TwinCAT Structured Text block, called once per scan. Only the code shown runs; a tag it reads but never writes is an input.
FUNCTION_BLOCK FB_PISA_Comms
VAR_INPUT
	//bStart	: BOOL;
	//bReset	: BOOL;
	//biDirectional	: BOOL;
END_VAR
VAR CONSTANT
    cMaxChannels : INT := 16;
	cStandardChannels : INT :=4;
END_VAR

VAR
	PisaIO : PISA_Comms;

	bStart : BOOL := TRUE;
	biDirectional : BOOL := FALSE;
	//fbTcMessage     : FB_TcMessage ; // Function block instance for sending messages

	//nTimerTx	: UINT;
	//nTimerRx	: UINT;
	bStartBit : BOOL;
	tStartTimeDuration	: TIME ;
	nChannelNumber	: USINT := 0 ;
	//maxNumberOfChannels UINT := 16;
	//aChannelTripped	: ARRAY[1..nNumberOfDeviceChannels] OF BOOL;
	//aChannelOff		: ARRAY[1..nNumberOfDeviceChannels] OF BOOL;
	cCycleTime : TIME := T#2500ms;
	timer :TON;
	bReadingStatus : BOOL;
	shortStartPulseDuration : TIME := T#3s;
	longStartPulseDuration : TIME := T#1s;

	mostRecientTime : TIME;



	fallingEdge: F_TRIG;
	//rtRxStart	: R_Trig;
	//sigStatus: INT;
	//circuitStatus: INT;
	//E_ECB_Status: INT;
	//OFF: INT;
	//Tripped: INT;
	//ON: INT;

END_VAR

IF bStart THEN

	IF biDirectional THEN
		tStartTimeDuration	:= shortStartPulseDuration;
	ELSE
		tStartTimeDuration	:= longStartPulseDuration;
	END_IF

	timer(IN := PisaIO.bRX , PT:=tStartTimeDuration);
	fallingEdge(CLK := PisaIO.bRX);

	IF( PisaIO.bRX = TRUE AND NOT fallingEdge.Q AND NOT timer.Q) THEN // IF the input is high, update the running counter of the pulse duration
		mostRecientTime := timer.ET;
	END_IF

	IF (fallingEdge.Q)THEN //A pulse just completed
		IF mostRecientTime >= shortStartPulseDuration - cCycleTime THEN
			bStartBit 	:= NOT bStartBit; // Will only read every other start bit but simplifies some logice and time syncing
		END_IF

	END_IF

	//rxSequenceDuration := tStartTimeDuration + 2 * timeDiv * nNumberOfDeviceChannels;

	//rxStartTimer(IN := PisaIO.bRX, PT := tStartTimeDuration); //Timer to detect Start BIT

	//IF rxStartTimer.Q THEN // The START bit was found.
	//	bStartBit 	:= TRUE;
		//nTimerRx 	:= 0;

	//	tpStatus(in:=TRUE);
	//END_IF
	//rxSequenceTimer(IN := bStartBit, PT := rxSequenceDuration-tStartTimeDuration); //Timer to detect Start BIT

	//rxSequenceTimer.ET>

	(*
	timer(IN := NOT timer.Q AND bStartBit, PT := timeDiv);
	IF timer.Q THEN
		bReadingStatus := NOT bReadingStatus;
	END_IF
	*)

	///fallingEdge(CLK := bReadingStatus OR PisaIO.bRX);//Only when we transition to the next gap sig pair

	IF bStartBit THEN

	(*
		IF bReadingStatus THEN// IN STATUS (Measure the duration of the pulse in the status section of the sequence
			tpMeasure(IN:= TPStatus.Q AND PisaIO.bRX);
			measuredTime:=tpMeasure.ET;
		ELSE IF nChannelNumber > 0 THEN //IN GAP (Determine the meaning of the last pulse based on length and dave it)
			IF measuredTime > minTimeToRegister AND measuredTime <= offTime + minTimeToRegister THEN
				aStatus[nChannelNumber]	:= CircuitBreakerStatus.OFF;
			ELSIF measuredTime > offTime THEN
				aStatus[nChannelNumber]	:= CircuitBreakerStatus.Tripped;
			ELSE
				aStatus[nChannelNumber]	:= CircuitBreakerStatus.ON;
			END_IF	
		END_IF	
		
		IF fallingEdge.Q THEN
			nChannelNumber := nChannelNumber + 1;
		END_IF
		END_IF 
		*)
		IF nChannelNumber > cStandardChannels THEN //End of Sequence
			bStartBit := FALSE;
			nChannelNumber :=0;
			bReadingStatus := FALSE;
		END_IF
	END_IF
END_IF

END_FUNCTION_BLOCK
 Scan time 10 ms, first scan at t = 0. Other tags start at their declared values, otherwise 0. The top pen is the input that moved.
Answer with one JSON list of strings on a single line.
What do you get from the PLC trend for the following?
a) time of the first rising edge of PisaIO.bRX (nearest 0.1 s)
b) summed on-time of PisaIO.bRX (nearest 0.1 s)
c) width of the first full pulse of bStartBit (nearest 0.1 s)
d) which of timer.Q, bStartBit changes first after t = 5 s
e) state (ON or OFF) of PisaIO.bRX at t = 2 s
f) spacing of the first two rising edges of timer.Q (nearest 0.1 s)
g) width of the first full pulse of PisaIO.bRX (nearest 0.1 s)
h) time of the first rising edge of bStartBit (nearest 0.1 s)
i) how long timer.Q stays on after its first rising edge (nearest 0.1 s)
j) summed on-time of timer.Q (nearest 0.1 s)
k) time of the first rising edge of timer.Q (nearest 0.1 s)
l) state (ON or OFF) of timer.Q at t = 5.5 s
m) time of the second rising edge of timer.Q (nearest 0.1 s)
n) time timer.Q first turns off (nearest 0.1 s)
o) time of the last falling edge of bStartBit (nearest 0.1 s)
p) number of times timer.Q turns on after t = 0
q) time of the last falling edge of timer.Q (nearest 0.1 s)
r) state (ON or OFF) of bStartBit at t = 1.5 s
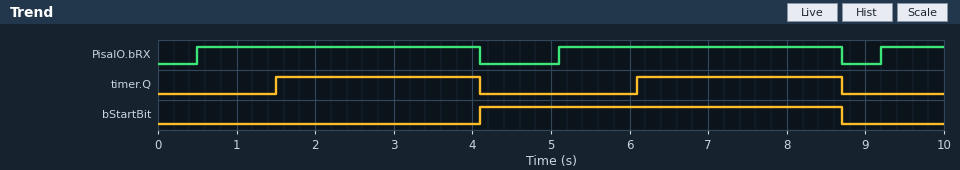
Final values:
["0.5 s", "8.0 s", "4.6 s", "timer.Q", "ON", "4.6 s", "3.6 s", "4.1 s", "2.6 s", "5.2 s", "1.5 s", "OFF", "6.1 s", "4.1 s", "8.7 s", "2", "8.7 s", "OFF"]
